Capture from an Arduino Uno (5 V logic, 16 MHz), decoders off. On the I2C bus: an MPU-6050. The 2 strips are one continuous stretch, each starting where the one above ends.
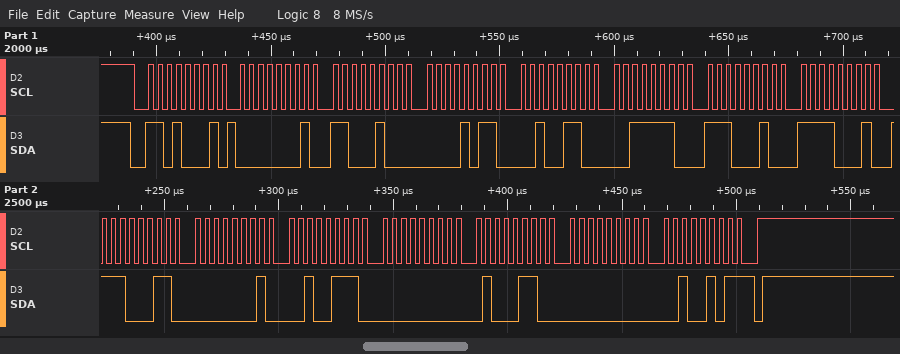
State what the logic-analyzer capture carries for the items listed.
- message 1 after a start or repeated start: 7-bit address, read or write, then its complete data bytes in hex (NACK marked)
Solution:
0x68 read: 01 C4 0B 26 3E E2 F1 E3 01 27 00 46 00 25 NACK
